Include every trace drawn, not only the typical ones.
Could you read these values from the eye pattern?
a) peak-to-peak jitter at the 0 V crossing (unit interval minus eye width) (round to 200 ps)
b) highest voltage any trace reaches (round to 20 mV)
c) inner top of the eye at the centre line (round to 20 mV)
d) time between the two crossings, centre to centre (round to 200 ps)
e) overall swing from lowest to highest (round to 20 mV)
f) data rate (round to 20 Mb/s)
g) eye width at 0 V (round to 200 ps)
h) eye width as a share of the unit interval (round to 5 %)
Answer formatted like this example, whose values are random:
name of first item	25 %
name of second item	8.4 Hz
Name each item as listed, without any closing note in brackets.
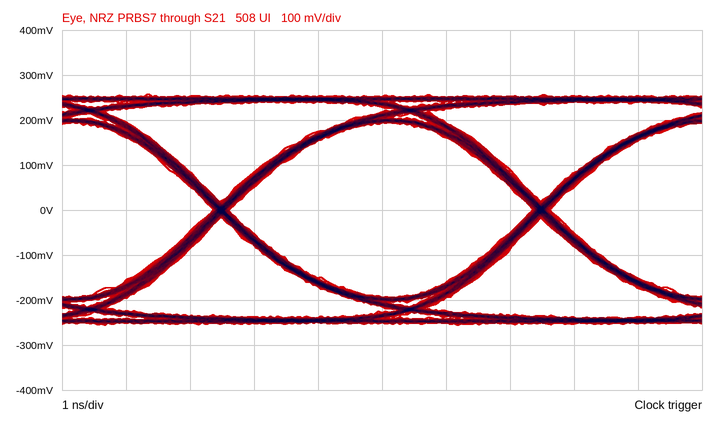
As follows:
peak-to-peak jitter at the 0 V crossing (unit interval minus eye width)	200 ps
highest voltage any trace reaches	260 mV
inner top of the eye at the centre line	200 mV
time between the two crossings, centre to centre	5.0 ns
overall swing from lowest to highest	520 mV
data rate	200 Mb/s
eye width at 0 V	4.8 ns
eye width as a share of the unit interval	95 %
